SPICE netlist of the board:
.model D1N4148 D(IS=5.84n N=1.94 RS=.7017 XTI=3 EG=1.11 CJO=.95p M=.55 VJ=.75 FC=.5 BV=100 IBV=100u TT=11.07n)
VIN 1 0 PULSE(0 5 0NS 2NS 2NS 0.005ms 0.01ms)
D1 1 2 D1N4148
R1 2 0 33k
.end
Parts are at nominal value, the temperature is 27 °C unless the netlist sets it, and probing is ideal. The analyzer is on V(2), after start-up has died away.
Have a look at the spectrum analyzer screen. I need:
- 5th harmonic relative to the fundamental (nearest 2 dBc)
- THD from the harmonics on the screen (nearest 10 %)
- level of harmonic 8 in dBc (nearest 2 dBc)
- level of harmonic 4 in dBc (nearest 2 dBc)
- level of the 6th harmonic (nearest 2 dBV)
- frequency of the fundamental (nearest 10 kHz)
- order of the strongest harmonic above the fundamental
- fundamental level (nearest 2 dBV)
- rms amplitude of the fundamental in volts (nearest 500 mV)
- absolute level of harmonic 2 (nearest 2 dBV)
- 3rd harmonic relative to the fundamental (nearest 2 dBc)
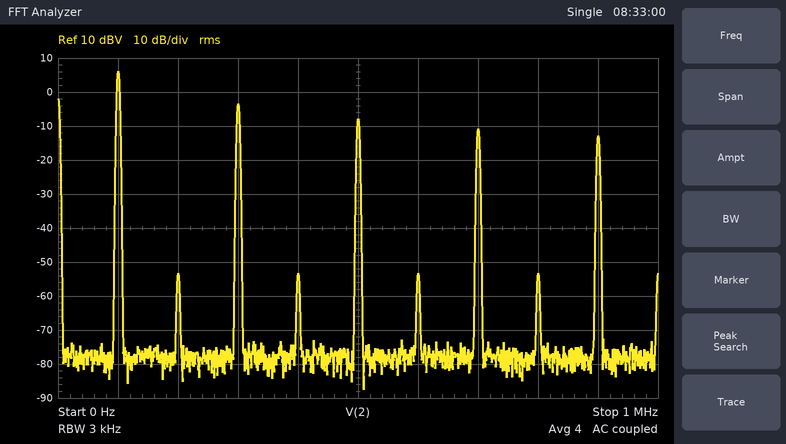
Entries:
-14 dBc
40 %
-60 dBc
-60 dBc
-54 dBV
100 kHz
3
6 dBV
2.0 V
-54 dBV
-10 dBc
